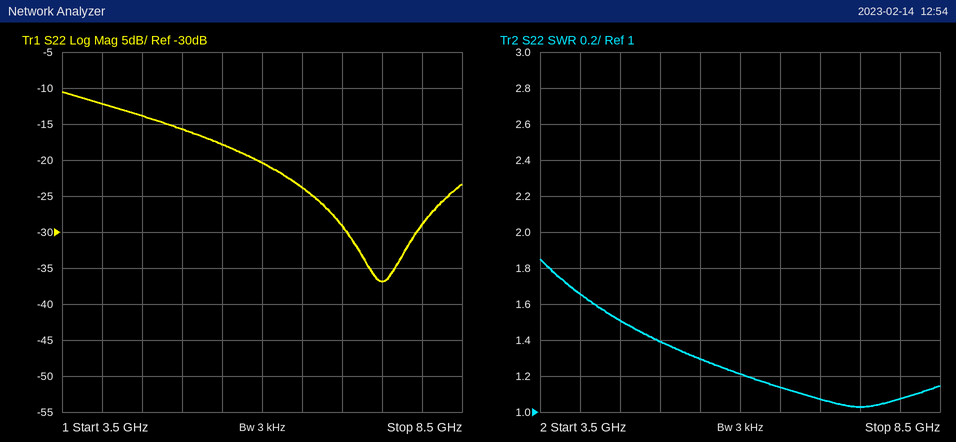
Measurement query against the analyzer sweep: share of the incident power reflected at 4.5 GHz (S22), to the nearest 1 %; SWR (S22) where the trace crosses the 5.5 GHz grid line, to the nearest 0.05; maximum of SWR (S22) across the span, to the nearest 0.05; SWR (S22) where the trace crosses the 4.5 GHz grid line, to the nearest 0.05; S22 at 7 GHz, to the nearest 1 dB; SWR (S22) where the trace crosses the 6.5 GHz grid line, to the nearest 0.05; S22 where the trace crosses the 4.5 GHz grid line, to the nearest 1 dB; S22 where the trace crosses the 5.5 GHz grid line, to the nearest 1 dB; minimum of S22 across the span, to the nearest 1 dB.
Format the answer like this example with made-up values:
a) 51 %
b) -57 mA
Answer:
a) 4 %
b) 1.30
c) 1.85
d) 1.50
e) -29 dB
f) 1.15
g) -14 dB
h) -18 dB
i) -37 dB
